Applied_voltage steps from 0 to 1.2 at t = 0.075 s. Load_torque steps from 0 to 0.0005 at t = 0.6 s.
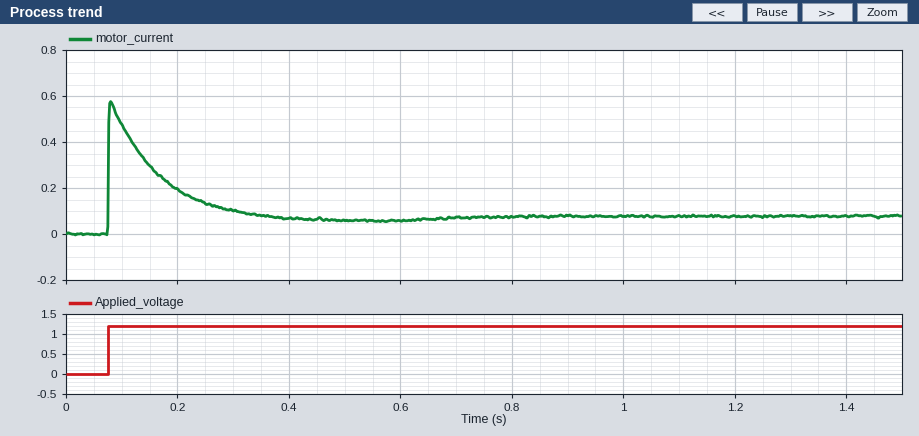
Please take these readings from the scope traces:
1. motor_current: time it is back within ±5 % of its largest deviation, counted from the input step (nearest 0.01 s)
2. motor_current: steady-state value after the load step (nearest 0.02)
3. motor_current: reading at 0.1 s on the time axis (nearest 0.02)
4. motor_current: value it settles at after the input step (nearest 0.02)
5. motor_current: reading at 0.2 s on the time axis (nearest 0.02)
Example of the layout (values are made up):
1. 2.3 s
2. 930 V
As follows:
1. 0.27 s
2. 0.08
3. 0.48
4. 0.06
5. 0.20
